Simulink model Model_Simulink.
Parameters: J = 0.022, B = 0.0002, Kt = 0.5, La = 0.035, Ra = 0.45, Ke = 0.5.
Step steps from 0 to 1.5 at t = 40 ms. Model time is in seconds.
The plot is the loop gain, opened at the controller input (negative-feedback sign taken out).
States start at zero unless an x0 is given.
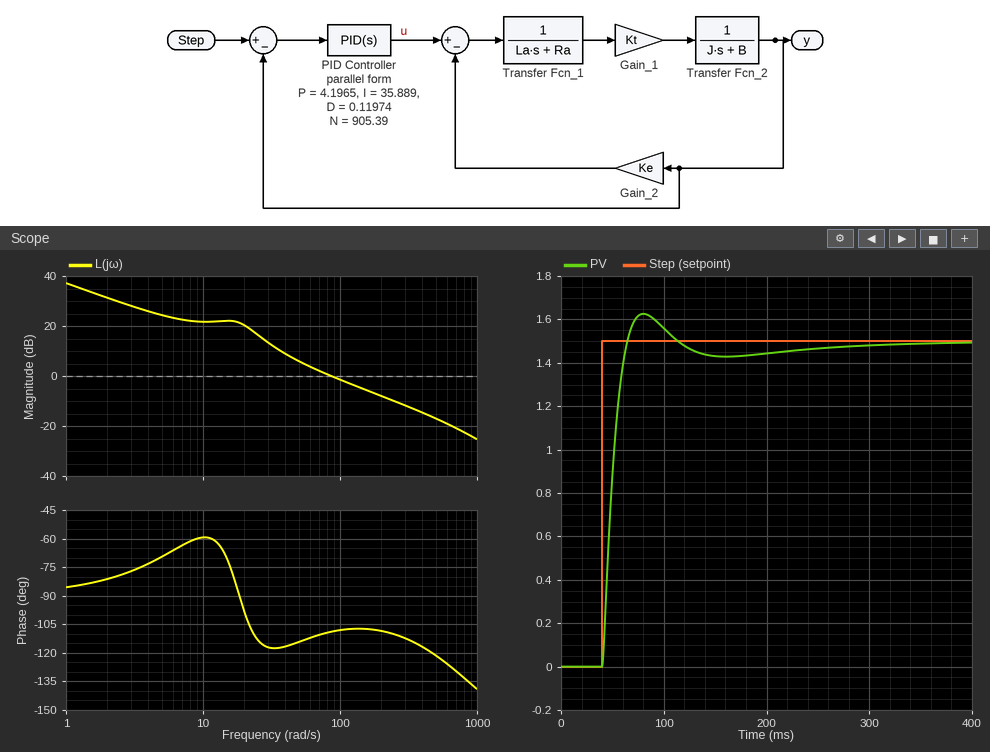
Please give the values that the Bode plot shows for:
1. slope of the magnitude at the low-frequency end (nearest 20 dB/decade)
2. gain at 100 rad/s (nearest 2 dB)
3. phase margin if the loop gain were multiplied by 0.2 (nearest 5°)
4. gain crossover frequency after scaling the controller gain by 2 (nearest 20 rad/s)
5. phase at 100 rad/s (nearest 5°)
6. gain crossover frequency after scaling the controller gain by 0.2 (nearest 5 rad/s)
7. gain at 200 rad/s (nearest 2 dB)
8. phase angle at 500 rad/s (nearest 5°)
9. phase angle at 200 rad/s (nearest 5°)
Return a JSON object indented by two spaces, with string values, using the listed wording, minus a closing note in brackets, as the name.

{
  "slope of the magnitude at the low-frequency end": "-20 dB/decade",
  "gain at 100 rad/s": "-2 dB",
  "phase margin if the loop gain were multiplied by 0.2": "65°",
  "gain crossover frequency after scaling the controller gain by 2": "160 rad/s",
  "phase at 100 rad/s": "-110°",
  "gain crossover frequency after scaling the controller gain by 0.2": "30 rad/s",
  "gain at 200 rad/s": "-8 dB",
  "phase angle at 500 rad/s": "-120°",
  "phase angle at 200 rad/s": "-110°"
}
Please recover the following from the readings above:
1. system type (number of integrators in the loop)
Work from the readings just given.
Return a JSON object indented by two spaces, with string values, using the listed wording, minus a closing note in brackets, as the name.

{
  "system type": "1"
}
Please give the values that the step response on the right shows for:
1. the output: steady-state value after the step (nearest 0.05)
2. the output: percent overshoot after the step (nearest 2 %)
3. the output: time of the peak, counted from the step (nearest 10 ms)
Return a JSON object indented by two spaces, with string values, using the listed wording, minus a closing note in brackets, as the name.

{
  "the output: steady-state value after the step": "1.50",
  "the output: percent overshoot after the step": "8 %",
  "the output: time of the peak, counted from the step": "40 ms"
}
